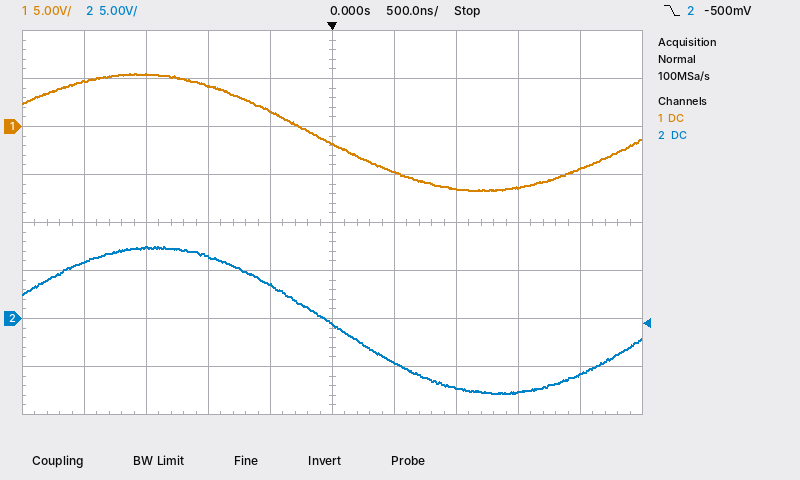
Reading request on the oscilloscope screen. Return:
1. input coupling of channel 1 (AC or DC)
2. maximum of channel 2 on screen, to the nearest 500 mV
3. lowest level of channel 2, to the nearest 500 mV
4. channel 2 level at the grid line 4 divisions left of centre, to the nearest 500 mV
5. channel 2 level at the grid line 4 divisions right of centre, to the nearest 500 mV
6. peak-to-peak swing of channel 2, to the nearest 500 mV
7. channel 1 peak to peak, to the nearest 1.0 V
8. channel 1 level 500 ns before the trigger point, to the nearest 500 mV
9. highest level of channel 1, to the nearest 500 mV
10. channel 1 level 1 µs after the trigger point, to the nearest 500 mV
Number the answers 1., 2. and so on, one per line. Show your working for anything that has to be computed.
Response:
1. DC
2. 7.5 V
3. -8.0 V
4. 6.0 V
5. -6.0 V
6. 7.5 V − (-8.0 V) = 15.5 V
7. 12.0 V
8. 1.5 V
9. 5.5 V
10. -6.5 V
